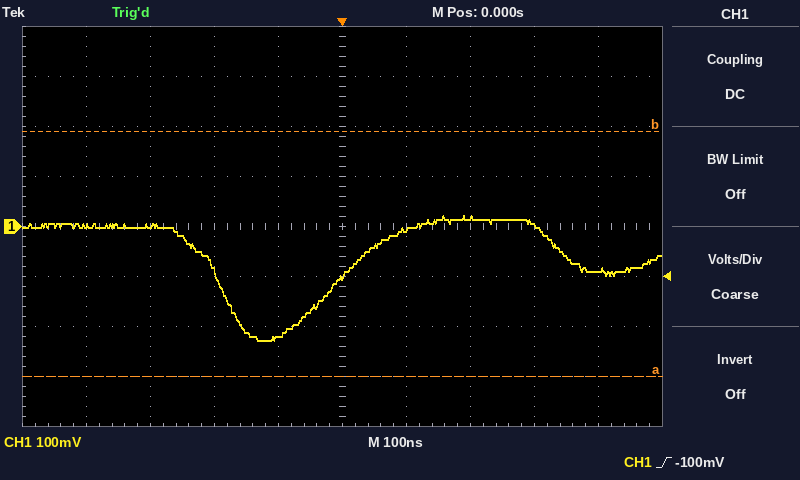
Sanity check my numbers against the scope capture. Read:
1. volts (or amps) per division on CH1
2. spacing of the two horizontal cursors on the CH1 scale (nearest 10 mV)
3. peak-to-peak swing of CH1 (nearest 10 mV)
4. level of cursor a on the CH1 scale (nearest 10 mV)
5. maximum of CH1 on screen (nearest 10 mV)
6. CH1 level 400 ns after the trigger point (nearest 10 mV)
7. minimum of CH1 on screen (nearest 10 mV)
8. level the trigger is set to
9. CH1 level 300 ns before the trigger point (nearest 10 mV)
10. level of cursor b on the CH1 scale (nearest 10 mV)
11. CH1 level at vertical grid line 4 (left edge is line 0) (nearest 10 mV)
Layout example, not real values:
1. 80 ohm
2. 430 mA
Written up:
1. 100 mV
2. 490 mV
3. 250 mV
4. -300 mV
5. 20 mV
6. -90 mV
7. -230 mV
8. -100 mV
9. 0 mV
10. 190 mV
11. -220 mV
